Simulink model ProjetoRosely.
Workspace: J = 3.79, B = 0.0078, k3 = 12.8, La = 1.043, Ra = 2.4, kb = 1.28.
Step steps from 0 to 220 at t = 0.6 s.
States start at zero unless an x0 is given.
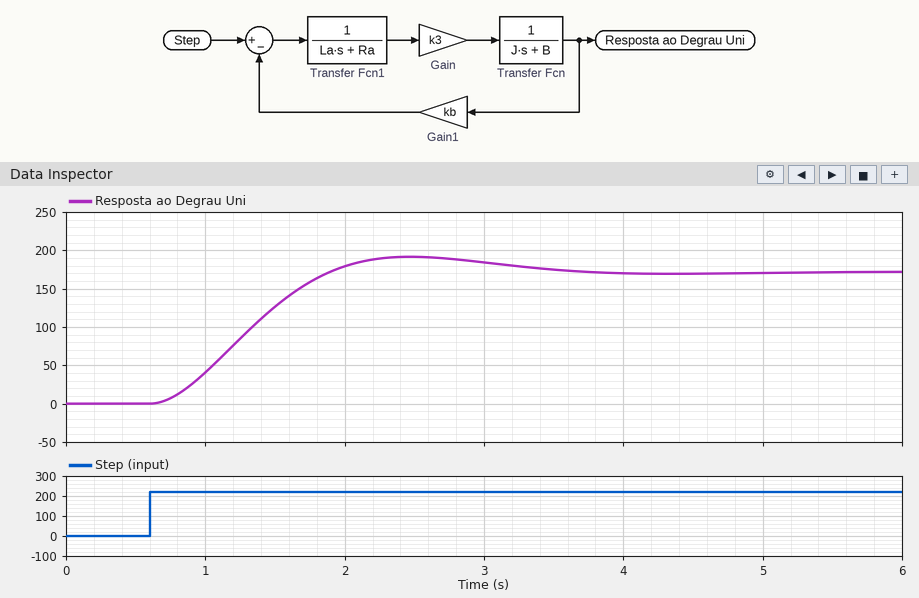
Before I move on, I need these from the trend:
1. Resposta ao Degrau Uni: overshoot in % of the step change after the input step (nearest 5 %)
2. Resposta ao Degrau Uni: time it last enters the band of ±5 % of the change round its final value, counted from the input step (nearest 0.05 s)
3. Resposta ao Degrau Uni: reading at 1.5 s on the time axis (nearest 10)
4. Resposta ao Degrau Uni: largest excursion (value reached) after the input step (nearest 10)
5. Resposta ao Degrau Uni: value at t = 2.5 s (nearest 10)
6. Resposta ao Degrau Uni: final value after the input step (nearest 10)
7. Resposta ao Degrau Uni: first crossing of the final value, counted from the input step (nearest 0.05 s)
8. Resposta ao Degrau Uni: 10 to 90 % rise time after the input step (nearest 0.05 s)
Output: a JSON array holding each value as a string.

["10 %", "2.60 s", "130", "190", "190", "170", "1.30 s", "0.85 s"]
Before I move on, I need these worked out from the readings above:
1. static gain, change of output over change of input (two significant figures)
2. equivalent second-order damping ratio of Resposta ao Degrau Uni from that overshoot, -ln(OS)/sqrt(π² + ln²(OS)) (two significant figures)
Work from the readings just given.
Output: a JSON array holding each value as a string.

["0.77", "0.59"]
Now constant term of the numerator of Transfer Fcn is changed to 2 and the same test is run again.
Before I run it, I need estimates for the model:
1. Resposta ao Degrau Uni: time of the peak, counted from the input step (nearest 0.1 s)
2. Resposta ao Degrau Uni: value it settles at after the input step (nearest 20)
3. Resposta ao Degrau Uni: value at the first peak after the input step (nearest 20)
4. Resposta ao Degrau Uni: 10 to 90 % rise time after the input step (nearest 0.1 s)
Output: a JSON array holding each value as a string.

["1.2 s", "180", "220", "0.5 s"]
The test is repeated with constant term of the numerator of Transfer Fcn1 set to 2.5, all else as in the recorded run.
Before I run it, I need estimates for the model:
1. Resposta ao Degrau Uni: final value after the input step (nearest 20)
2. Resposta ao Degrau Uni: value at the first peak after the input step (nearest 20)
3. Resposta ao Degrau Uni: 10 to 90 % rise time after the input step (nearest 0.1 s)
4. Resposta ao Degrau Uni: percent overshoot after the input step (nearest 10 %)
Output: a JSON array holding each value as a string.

["180", "220", "0.4 s", "30 %"]
